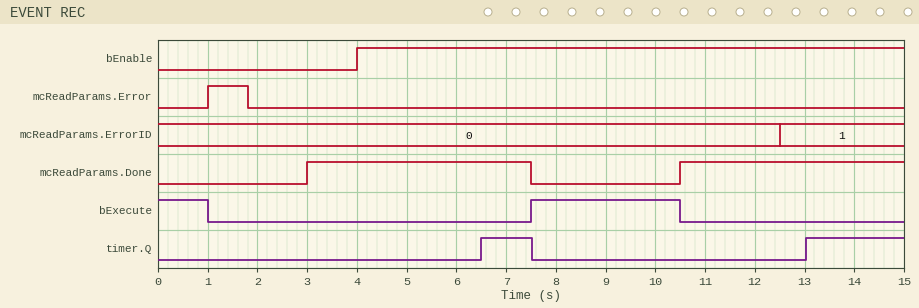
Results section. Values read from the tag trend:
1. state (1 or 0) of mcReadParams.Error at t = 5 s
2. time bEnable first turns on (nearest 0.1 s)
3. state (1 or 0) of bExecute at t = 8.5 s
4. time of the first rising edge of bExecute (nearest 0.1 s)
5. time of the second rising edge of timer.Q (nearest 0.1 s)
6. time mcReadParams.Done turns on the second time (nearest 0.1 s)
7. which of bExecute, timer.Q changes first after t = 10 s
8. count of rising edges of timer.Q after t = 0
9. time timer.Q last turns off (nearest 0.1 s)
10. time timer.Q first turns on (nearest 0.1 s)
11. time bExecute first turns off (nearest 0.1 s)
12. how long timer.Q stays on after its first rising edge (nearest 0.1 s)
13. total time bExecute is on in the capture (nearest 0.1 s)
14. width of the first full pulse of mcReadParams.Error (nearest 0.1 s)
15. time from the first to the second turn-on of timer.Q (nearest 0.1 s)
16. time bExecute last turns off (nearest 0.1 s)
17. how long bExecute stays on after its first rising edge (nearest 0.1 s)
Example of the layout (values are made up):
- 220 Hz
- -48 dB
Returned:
- 0
- 4.0 s
- 1
- 7.5 s
- 13.0 s
- 10.5 s
- bExecute
- 2
- 7.5 s
- 6.5 s
- 1.0 s
- 1.0 s
- 4.0 s
- 0.8 s
- 6.5 s
- 10.5 s
- 3.0 s
